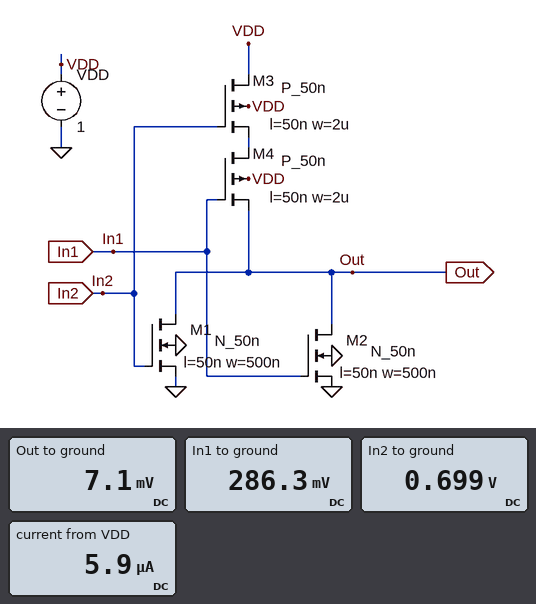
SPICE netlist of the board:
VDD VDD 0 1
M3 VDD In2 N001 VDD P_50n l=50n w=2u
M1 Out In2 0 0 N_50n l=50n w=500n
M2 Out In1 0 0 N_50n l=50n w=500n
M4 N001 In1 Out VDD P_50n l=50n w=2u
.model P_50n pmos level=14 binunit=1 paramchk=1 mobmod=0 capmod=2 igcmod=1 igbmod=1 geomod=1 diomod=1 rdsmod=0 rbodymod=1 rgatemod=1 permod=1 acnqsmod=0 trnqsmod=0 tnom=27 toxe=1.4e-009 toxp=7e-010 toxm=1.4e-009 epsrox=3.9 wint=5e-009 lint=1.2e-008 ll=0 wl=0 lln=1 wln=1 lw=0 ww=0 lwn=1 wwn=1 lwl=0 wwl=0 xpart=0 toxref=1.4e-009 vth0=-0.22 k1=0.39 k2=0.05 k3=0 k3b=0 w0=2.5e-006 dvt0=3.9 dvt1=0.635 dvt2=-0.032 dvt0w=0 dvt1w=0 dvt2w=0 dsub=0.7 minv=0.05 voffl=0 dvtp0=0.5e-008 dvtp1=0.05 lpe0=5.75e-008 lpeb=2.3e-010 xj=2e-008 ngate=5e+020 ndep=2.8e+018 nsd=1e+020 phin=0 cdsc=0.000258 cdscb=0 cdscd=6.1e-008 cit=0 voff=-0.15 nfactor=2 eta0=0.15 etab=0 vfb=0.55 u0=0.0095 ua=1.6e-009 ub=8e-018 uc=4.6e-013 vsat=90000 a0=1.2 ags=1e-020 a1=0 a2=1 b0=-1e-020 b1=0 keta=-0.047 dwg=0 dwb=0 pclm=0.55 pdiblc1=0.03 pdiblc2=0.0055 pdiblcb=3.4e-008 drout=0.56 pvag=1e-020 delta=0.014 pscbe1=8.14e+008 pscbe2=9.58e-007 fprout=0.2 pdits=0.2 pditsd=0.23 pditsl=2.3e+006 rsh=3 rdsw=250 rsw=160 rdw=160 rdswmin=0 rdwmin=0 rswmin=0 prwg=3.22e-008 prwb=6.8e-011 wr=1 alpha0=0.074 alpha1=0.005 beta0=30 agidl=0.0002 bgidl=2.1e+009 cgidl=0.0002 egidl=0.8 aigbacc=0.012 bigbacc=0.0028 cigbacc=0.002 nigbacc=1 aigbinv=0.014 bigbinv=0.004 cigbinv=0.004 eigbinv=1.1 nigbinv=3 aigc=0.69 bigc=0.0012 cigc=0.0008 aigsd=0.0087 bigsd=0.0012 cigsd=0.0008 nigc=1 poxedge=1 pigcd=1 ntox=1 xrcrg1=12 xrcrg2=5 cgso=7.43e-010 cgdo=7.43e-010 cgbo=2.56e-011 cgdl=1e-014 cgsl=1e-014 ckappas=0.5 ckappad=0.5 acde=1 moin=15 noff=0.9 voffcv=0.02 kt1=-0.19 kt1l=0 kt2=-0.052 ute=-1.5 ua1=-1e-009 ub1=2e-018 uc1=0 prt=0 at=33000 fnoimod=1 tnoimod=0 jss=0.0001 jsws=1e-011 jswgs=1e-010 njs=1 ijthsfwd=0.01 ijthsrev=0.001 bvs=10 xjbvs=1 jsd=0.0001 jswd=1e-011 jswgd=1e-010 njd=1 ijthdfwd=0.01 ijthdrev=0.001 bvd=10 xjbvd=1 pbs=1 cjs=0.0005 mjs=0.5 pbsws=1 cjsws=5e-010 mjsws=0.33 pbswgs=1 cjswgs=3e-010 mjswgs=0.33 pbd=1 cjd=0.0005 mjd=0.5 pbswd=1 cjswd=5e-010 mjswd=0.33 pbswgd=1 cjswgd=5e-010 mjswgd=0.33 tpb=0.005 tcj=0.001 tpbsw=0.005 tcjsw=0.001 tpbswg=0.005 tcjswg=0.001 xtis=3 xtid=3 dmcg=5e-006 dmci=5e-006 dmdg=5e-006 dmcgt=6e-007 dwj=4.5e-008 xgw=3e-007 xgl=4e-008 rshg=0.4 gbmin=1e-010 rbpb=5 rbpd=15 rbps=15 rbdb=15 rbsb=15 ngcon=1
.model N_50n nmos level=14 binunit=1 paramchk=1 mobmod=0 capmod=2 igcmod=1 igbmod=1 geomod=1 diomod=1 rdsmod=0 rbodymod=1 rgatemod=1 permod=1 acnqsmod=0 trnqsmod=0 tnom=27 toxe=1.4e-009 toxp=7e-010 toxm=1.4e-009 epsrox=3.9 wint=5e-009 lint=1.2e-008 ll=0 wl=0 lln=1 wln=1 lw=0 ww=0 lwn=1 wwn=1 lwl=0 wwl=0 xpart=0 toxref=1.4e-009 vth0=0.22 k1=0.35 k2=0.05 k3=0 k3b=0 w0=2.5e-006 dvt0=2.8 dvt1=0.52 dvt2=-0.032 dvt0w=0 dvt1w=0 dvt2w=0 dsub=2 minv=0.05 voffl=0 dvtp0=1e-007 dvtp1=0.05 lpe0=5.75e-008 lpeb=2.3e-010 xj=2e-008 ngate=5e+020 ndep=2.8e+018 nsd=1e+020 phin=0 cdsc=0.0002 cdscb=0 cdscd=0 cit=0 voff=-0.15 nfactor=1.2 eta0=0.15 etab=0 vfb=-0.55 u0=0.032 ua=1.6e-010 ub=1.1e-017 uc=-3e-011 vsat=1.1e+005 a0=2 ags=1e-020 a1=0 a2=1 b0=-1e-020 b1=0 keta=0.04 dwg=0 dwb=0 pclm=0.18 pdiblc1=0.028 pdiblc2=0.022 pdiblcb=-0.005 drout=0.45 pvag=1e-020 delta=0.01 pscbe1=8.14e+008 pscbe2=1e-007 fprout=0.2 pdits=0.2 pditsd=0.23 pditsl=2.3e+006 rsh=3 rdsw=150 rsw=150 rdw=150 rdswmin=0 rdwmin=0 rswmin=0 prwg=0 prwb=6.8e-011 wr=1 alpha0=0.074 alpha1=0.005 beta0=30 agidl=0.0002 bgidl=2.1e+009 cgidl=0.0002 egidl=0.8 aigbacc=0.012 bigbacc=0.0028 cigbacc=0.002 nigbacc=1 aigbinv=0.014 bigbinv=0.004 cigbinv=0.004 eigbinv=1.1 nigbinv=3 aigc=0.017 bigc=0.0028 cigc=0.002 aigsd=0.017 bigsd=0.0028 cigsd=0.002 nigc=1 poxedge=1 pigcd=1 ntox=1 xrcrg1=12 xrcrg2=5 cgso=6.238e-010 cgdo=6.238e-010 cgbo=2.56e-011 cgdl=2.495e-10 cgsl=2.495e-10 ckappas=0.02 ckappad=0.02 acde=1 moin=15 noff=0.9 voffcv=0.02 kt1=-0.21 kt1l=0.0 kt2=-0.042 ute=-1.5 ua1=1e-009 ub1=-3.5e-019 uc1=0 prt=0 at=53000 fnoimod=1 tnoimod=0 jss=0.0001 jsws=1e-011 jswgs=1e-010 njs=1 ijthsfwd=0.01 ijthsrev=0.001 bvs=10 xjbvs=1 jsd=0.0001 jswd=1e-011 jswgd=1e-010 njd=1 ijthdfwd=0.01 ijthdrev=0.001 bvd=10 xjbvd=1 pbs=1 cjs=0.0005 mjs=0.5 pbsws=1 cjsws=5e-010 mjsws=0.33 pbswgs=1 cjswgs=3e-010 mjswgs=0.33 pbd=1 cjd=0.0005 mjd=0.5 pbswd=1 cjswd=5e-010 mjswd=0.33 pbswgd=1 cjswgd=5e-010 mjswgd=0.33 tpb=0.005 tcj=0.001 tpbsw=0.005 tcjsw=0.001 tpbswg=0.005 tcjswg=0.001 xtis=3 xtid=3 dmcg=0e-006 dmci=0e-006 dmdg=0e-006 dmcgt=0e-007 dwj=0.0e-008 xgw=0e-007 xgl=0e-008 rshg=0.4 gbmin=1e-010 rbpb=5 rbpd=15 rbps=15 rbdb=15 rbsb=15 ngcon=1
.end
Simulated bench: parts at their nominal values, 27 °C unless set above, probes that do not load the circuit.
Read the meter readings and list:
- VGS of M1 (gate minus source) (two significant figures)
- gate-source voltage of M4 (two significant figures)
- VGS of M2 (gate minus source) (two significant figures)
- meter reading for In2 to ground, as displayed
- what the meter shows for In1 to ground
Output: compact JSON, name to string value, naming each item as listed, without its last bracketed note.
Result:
{"VGS of M1 (gate minus source)": "700 mV", "gate-source voltage of M4": "280 mV", "VGS of M2 (gate minus source)": "290 mV", "meter reading for In2 to ground, as displayed": "0.699 V", "what the meter shows for In1 to ground": "286.3 mV"}
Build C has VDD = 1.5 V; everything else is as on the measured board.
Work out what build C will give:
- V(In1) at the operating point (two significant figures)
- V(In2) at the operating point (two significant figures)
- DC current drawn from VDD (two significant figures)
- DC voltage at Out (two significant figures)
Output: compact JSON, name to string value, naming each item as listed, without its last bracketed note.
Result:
{"V(In1) at the operating point": "520 mV", "V(In2) at the operating point": "1.0 V", "DC current drawn from VDD": "89 µA", "DC voltage at Out": "67 mV"}
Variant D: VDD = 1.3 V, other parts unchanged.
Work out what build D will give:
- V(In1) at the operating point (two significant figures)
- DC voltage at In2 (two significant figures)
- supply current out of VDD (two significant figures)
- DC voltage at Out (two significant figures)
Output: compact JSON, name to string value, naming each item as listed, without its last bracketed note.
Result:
{"V(In1) at the operating point": "420 mV", "DC voltage at In2": "880 mV", "supply current out of VDD": "38 µA", "DC voltage at Out": "34 mV"}
